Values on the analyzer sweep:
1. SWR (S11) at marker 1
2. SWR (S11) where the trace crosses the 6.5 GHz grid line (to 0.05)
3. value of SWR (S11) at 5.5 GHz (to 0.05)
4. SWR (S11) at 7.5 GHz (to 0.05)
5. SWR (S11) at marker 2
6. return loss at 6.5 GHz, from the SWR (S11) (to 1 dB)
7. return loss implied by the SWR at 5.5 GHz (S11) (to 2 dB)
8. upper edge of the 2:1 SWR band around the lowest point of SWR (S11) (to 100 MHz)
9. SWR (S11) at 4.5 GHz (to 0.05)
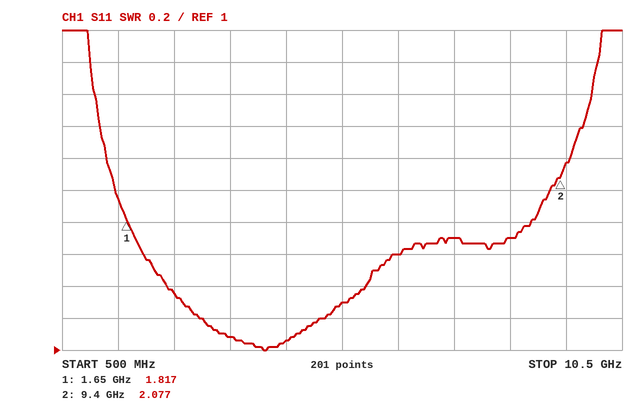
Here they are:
1.817
1.60
1.30
1.70
2.077
13 dB
18 dB
9.2 GHz
1.05
